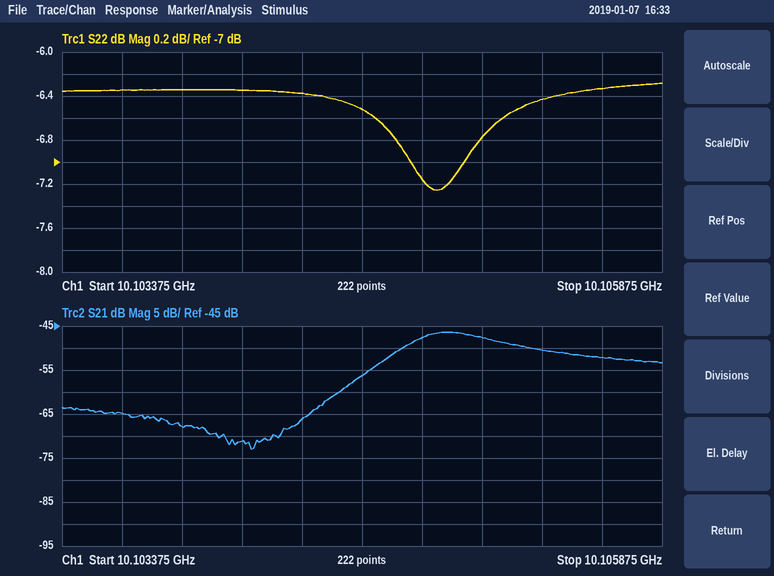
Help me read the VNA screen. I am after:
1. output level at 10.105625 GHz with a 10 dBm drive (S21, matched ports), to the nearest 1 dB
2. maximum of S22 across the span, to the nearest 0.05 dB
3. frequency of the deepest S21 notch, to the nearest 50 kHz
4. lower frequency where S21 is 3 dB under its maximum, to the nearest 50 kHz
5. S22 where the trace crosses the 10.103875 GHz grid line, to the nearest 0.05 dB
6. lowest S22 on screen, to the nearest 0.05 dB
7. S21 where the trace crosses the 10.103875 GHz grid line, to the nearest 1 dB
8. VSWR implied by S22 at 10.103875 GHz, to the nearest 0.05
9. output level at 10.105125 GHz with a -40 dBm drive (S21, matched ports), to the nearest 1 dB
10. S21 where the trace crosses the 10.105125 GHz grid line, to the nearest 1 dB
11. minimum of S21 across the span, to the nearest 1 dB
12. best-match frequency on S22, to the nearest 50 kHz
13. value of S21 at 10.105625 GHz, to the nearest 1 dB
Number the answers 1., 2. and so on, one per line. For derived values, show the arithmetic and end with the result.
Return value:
1. 10 dBm + (-52 dB) = -42 dBm
2. -6.30 dB
3. 10.10415 GHz
4. 10.10480 GHz
5. -6.35 dB
6. -7.25 dB
7. -68 dB
8. |Γ| = 10^(-6.35/20) = 0.4814; VSWR = (1 + 0.4814)/(1 − 0.4814) ≈ 2.86, so 2.85 to the nearest 0.05
9. -40 dBm + (-48 dB) = -88 dBm
10. -48 dB
11. -73 dB
12. 10.10495 GHz
13. -52 dB
